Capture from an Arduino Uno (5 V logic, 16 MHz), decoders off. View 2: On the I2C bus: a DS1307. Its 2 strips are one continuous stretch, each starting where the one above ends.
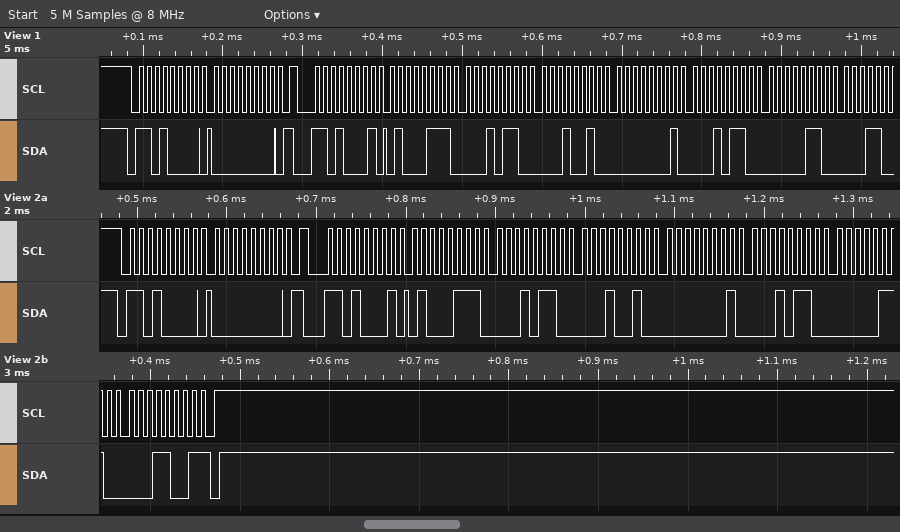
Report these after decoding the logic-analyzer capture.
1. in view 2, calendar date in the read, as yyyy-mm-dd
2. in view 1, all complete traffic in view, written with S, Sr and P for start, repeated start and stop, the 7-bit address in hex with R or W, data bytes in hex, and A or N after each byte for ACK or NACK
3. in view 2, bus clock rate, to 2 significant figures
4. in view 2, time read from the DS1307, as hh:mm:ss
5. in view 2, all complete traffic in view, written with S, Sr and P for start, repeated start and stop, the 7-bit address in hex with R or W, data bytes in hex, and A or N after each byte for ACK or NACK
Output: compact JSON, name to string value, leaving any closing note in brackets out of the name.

{"in view 2, calendar date in the read, as yyyy-mm-dd": "2019-06-16", "in view 1, all complete traffic in view, written with S, Sr and P for start, repeated start and stop, the 7-bit address in hex with R or W, data bytes in hex, and A or N after each byte for ACK or NACK": "S 68W A 00 A Sr 68R A 47 A 16 A 12 A 01 A 16 A 06 A", "in view 2, bus clock rate, to 2 significant figures": "100 kHz", "in view 2, time read from the DS1307, as hh:mm:ss": "12:16:47", "in view 2, all complete traffic in view, written with S, Sr and P for start, repeated start and stop, the 7-bit address in hex with R or W, data bytes in hex, and A or N after each byte for ACK or NACK": "S 68W A 00 A Sr 68R A 47 A 16 A 12 A 01 A 16 A 06 A 19 N P"}
